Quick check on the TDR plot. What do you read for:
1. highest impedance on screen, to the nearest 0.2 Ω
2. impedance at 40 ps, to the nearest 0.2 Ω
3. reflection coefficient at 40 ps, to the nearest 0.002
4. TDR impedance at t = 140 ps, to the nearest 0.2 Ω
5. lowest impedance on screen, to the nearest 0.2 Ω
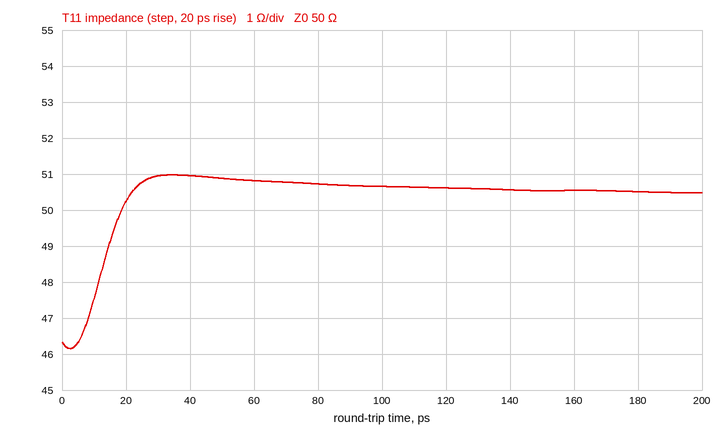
51.0 Ω
51.0 Ω
+0.010
50.6 Ω
46.2 Ω
